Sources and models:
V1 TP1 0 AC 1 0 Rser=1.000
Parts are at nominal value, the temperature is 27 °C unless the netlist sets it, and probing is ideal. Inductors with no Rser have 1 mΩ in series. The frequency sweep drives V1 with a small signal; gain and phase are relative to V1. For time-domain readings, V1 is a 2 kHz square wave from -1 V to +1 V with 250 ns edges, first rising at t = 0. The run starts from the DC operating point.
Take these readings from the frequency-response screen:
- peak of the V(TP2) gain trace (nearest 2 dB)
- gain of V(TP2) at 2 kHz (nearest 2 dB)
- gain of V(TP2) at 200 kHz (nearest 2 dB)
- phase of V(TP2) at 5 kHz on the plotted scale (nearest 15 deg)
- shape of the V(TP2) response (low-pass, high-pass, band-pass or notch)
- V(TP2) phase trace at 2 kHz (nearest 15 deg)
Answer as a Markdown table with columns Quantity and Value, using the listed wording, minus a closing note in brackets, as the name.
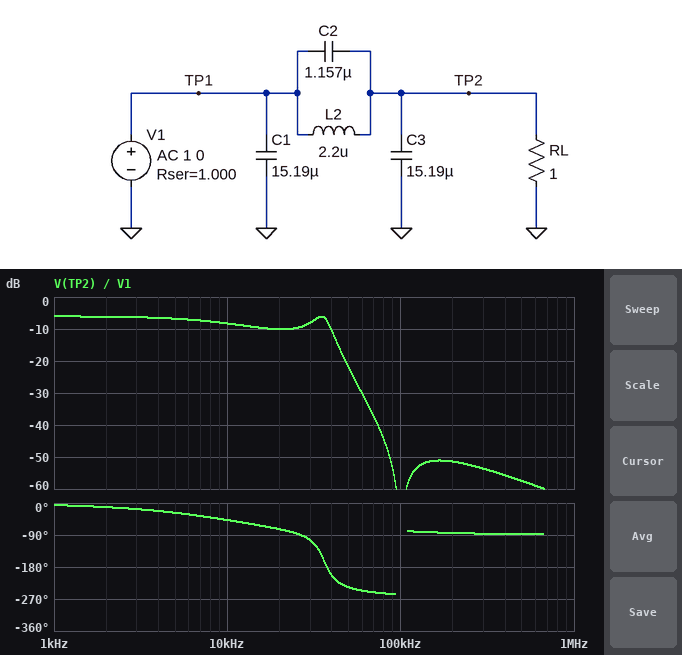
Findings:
| Quantity | Value |
|---|---|
| peak of the V(TP2) gain trace | -6 dB |
| gain of V(TP2) at 2 kHz | -6 dB |
| gain of V(TP2) at 200 kHz | -52 dB |
| phase of V(TP2) at 5 kHz on the plotted scale | -30 deg |
| shape of the V(TP2) response | low-pass |
| V(TP2) phase trace at 2 kHz | -15 deg |
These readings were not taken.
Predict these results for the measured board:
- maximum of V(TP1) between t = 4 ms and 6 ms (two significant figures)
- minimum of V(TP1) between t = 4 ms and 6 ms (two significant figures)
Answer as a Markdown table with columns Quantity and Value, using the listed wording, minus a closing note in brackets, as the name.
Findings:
| Quantity | Value |
|---|---|
| maximum of V(TP1) between t = 4 ms and 6 ms | 530 mV |
| minimum of V(TP1) between t = 4 ms and 6 ms | -530 mV |
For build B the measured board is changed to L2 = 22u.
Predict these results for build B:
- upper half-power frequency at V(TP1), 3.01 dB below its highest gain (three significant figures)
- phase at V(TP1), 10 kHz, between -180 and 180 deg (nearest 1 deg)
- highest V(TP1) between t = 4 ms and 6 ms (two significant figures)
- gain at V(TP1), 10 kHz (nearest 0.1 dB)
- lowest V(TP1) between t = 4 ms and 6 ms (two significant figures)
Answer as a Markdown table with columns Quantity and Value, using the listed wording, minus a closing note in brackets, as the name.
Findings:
| Quantity | Value |
|---|---|
| upper half-power frequency at V(TP1), 3.01 dB below its highest gain | 18.8 kHz |
| phase at V(TP1), 10 kHz, between -180 and 180 deg | -8 deg |
| highest V(TP1) between t = 4 ms and 6 ms | 730 mV |
| gain at V(TP1), 10 kHz | -2.9 dB |
| lowest V(TP1) between t = 4 ms and 6 ms | -730 mV |
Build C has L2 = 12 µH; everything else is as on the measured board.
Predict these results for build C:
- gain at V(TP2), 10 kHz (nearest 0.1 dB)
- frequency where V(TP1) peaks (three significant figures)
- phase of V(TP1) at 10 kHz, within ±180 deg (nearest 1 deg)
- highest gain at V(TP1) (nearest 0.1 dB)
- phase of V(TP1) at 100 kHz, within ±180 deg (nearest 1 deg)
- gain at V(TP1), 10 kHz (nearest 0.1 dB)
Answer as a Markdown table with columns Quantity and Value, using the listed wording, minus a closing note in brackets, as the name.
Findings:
| Quantity | Value |
|---|---|
| gain at V(TP2), 10 kHz | -6.2 dB |
| frequency where V(TP1) peaks | 16.3 kHz |
| phase of V(TP1) at 10 kHz, within ±180 deg | -3 deg |
| highest gain at V(TP1) | -3.1 dB |
| phase of V(TP1) at 100 kHz, within ±180 deg | -84 deg |
| gain at V(TP1), 10 kHz | -7.8 dB |
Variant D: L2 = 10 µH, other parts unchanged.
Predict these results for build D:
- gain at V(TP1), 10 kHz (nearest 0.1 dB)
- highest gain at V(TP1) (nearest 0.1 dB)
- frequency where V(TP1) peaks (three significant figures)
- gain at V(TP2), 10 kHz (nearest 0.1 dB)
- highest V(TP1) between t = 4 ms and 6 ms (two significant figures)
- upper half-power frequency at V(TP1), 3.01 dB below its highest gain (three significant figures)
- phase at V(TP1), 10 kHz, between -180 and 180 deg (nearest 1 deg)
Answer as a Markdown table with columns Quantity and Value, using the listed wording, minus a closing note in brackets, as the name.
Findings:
| Quantity | Value |
|---|---|
| gain at V(TP1), 10 kHz | -8.9 dB |
| highest gain at V(TP1) | -3.3 dB |
| frequency where V(TP1) peaks | 17.8 kHz |
| gain at V(TP2), 10 kHz | -6.5 dB |
| highest V(TP1) between t = 4 ms and 6 ms | 560 mV |
| upper half-power frequency at V(TP1), 3.01 dB below its highest gain | 24.6 kHz |
| phase at V(TP1), 10 kHz, between -180 and 180 deg | -9 deg |
